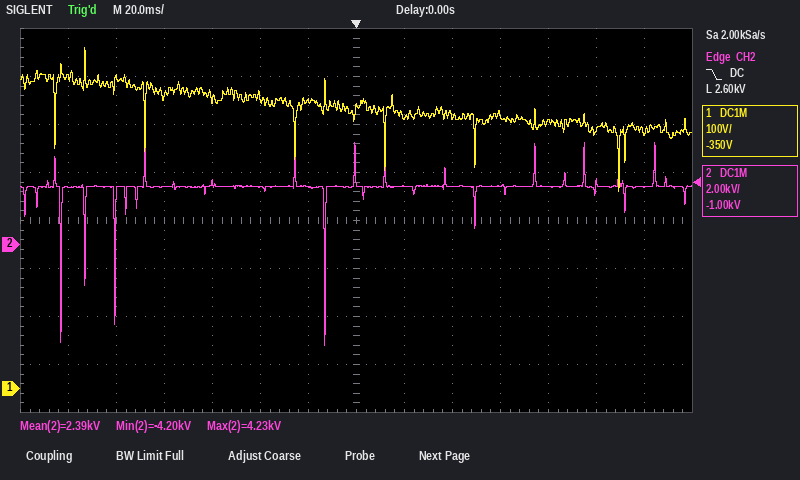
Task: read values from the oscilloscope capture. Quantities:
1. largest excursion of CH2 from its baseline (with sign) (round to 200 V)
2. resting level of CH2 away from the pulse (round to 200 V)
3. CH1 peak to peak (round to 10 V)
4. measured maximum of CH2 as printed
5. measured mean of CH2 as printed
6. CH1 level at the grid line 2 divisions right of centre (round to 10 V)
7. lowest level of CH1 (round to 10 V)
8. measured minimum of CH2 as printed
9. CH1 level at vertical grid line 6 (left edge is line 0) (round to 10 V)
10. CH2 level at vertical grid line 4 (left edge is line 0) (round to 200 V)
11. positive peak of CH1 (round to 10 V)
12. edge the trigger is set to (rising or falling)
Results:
-6.6 kV
2.4 kV
300 V
4.23 kV
2.39 kV
570 V
410 V
-4.20 kV
600 V
2.6 kV
710 V
falling
